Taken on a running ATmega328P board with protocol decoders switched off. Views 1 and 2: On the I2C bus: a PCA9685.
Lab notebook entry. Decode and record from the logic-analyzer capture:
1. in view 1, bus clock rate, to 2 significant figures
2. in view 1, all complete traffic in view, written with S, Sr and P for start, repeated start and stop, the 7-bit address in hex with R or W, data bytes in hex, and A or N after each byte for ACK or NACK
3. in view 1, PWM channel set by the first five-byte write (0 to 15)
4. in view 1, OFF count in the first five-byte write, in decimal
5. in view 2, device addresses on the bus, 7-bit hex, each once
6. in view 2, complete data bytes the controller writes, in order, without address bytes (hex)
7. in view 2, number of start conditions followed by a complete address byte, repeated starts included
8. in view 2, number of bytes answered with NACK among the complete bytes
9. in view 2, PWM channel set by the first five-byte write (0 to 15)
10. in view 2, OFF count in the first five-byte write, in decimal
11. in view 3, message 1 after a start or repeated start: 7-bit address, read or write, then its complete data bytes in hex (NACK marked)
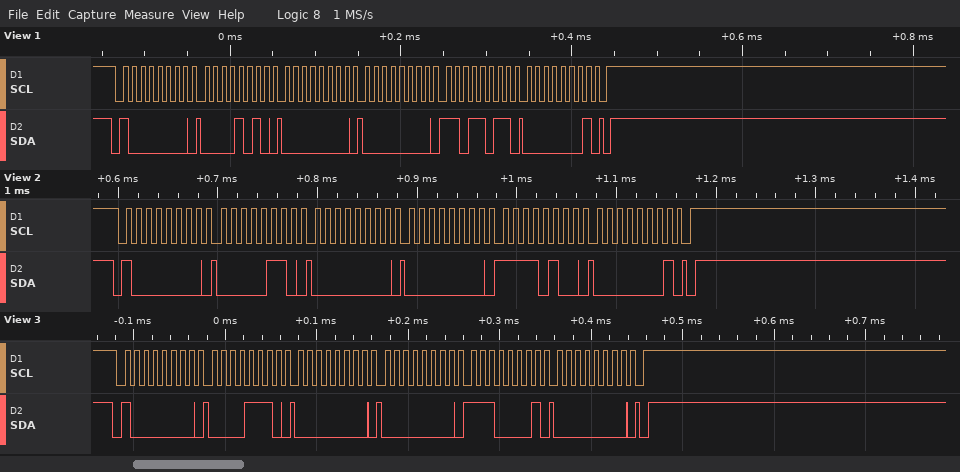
100 kHz
S 40W A 0A A 00 A 00 A DB A 01 A P
1
475
0x40
06 00 00 F4 01
1
0
0
500
0x40 write: 0E 00 00 E1 00
